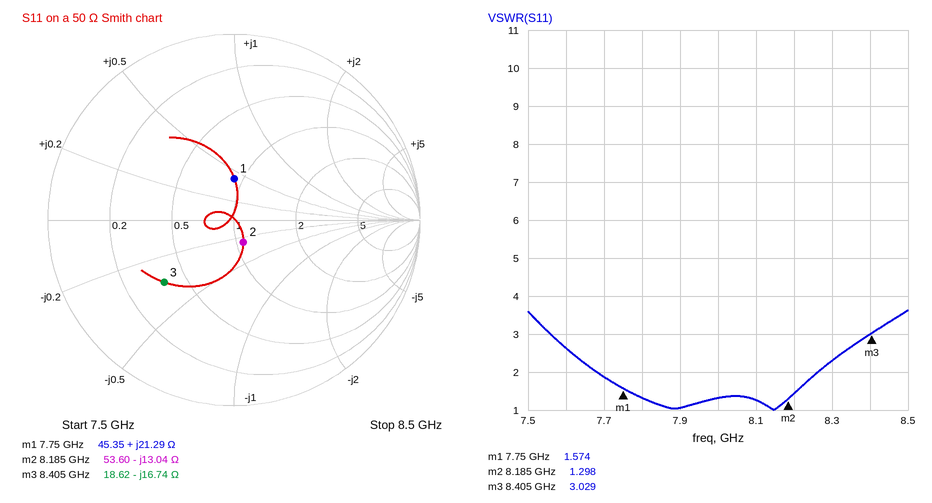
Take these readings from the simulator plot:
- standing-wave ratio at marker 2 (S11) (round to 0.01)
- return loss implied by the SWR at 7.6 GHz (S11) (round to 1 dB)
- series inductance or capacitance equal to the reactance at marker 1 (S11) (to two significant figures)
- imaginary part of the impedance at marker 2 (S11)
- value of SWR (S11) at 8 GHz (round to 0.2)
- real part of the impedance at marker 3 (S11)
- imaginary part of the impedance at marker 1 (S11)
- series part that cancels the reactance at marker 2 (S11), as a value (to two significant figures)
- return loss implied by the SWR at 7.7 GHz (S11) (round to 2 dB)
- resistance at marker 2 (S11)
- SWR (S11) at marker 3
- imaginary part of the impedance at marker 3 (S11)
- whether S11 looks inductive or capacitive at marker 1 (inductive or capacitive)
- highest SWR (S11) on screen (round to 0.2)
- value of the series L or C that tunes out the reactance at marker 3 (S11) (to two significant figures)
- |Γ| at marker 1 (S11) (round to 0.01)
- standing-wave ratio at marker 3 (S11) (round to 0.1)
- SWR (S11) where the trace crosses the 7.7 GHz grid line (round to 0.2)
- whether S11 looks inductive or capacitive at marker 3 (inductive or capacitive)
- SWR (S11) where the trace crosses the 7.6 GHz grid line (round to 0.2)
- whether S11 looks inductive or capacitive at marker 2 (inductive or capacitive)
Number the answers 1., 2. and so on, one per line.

1. 1.30
2. 7 dB
3. 440 pH
4. -13.04 Ω
5. 1.4
6. 18.62 Ω
7. +21.29 Ω
8. 250 pH
9. 10 dB
10. 53.60 Ω
11. 3.029
12. -16.74 Ω
13. inductive
14. 3.6
15. 320 pH
16. 0.22
17. 3.0
18. 1.8
19. capacitive
20. 2.6
21. capacitive
